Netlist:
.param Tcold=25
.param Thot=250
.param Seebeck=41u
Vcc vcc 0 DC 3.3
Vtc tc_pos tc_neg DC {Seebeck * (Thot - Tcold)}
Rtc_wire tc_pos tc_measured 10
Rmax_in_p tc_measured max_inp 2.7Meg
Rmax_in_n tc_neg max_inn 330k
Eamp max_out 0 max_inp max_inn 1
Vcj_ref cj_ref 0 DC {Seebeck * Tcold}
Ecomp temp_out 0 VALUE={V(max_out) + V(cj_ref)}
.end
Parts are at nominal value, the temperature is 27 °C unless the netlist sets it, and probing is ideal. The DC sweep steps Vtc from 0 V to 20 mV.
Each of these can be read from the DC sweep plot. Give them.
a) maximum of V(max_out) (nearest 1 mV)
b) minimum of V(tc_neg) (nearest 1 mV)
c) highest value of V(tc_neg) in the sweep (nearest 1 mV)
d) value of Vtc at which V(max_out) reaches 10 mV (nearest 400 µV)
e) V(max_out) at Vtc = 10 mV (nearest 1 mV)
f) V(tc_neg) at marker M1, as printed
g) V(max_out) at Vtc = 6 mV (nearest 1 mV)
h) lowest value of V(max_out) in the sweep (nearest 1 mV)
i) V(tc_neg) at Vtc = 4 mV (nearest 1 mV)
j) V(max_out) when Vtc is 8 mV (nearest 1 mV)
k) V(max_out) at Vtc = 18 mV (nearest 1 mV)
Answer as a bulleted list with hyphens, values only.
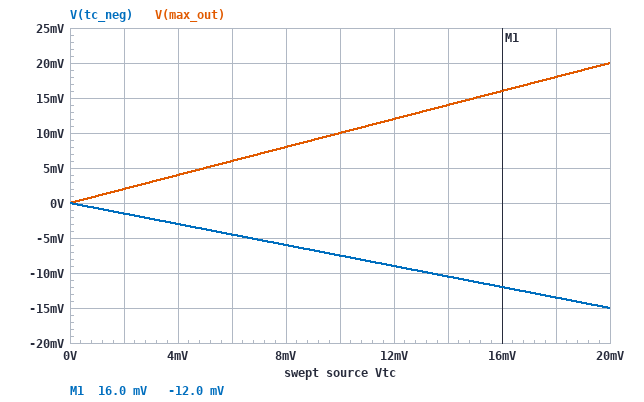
- 20 mV
- -15 mV
- 0 V
- 10.0 mV
- 10 mV
- -12.0 mV
- 6 mV
- 0 V
- -3 mV
- 8 mV
- 18 mV
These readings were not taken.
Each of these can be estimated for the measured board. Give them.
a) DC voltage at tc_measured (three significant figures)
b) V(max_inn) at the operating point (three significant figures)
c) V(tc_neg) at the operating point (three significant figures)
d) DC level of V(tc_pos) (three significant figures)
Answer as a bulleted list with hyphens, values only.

- 2.31 mV
- -6.92 mV
- -6.92 mV
- 2.31 mV
